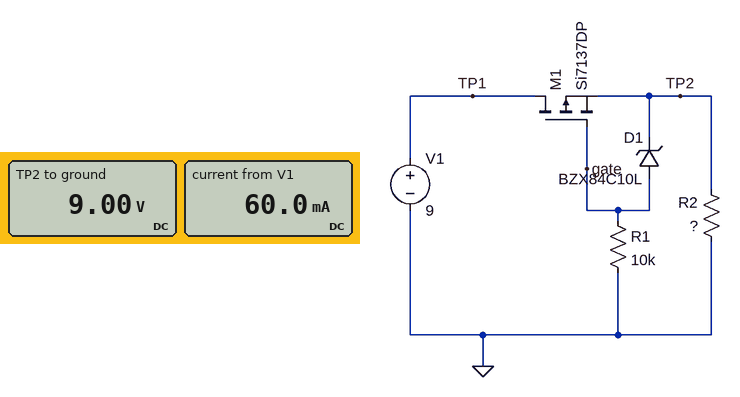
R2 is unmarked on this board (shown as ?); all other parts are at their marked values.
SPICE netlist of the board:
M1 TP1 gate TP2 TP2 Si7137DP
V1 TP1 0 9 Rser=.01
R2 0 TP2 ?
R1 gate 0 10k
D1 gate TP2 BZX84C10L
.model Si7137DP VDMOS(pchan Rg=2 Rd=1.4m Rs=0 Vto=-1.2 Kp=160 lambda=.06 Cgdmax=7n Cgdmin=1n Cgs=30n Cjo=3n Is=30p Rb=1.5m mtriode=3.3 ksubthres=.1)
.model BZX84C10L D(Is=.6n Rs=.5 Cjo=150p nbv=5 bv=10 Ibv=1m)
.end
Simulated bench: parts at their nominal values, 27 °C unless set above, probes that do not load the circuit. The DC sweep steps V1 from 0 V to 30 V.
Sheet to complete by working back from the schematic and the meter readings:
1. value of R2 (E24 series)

150 Ω
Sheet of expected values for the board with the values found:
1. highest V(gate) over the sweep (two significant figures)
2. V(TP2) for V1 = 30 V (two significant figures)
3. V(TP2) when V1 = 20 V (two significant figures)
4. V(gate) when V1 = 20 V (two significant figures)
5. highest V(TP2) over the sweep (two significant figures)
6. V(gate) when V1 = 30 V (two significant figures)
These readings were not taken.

20 V
30 V
20 V
10 V
30 V
20 V
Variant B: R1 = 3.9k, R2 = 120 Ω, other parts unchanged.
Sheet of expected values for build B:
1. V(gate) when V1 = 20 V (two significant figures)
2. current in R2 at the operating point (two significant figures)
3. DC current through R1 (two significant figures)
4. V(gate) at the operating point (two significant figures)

9.9 V
75 mA
430 nA
1.7 mV
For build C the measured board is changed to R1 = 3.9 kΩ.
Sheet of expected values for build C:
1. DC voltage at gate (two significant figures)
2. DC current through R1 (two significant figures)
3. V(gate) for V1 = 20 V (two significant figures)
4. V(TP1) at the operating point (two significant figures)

1.7 mV
430 nA
9.9 V
9.0 V
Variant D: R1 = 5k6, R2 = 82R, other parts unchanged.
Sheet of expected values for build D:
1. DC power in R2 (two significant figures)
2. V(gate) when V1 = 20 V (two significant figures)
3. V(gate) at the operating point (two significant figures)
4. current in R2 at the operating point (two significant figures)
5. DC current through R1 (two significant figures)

990 mW
9.9 V
2.4 mV
110 mA
430 nA
